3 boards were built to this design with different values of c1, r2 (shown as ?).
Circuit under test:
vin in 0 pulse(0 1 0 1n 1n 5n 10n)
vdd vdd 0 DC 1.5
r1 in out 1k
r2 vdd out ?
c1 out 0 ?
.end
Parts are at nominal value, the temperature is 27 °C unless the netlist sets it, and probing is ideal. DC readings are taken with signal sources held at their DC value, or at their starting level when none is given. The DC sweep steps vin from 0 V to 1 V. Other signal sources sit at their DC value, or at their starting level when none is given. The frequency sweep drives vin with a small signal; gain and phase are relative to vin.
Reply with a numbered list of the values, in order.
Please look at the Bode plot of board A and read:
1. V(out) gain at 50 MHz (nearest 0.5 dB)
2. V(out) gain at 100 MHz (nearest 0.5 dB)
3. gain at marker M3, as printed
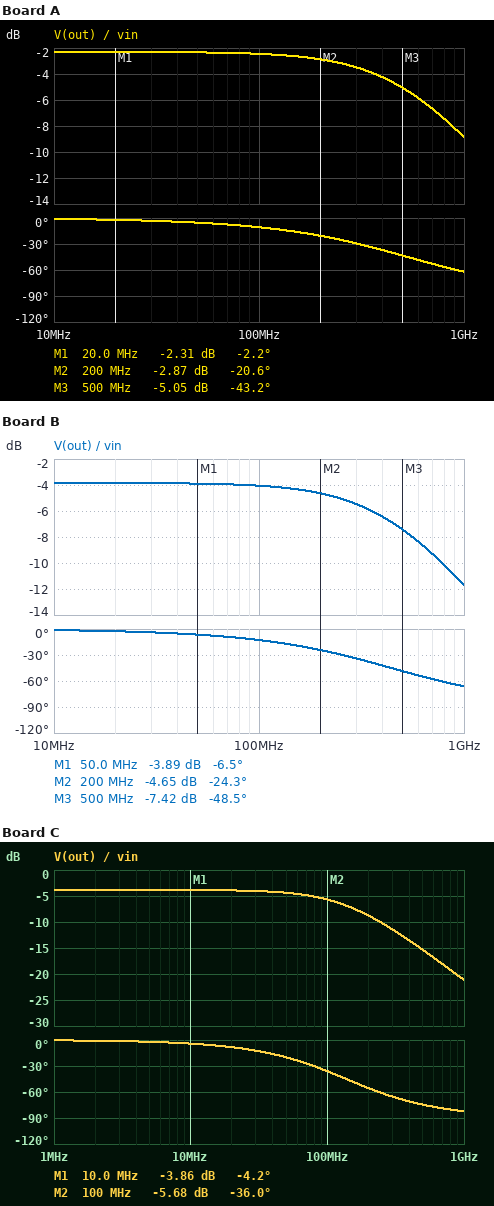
1. -2.5 dB
2. -2.5 dB
3. -5.05 dB
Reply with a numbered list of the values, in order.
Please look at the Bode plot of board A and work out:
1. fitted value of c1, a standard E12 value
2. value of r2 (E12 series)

1. 390 fF
2. 3.3 kΩ
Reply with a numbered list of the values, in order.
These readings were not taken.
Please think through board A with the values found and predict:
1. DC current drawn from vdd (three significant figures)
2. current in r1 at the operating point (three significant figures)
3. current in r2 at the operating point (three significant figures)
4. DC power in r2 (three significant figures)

1. 349 µA
2. 349 µA
3. 349 µA
4. 402 µW
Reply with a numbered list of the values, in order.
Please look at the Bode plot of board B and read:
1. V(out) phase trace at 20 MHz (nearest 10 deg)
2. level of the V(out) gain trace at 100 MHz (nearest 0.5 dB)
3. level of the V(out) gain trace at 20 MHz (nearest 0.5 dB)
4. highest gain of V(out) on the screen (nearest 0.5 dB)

1. 0 deg
2. -4.0 dB
3. -4.0 dB
4. -4.0 dB
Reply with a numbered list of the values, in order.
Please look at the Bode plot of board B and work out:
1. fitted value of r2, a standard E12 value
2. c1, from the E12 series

1. 1.8 kΩ
2. 560 fF
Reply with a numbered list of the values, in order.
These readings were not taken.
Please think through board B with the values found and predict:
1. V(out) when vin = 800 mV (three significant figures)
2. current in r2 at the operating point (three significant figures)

1. 1.05 V
2. 536 µA
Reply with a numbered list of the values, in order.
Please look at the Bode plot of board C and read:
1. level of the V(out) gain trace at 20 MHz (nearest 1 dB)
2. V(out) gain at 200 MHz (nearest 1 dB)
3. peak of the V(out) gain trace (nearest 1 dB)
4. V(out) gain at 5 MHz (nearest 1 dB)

1. -4 dB
2. -9 dB
3. -4 dB
4. -4 dB
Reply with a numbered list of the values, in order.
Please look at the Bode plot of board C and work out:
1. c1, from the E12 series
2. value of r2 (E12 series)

1. 1.8 pF
2. 1.8 kΩ
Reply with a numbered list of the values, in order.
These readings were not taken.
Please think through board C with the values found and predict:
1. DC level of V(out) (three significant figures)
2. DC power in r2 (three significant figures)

1. 536 mV
2. 517 µW
